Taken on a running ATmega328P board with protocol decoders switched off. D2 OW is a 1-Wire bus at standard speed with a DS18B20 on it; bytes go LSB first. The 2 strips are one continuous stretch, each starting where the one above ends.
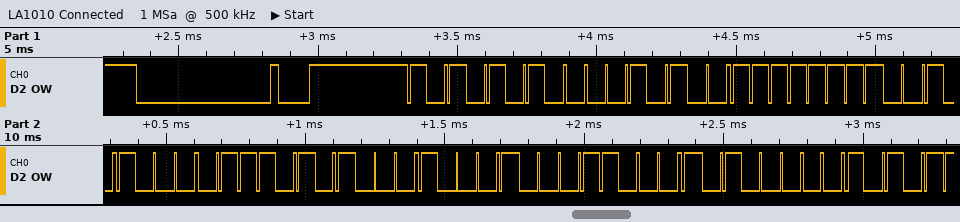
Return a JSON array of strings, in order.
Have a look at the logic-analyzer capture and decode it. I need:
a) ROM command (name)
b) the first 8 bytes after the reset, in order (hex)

["Match ROM", "55 28 FF 14 AE 88 18 05"]
